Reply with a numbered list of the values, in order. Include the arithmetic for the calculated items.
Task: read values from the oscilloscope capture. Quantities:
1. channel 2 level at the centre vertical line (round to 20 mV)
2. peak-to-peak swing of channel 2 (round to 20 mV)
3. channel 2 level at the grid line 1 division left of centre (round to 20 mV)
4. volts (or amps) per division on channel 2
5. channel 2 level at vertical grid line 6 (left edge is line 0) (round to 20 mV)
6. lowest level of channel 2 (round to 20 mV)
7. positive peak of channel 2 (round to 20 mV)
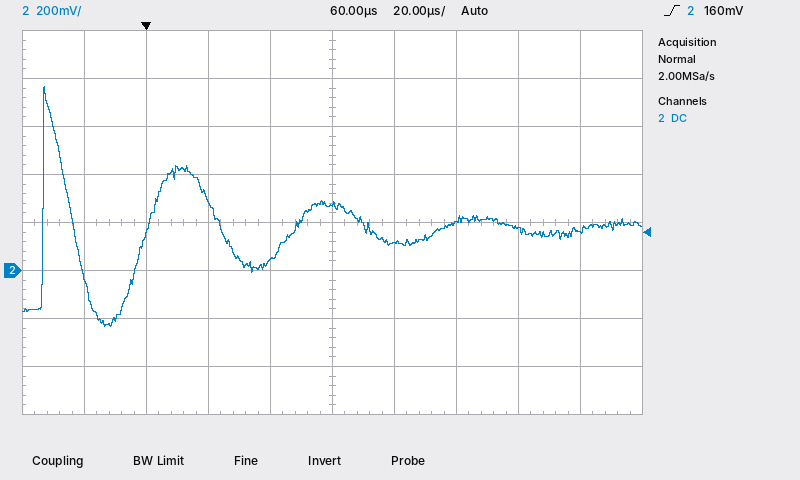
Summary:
1. 280 mV
2. 760 mV − (-240 mV) = 1.00 V
3. 40 mV
4. 200 mV
5. 120 mV
6. -240 mV
7. 760 mV
